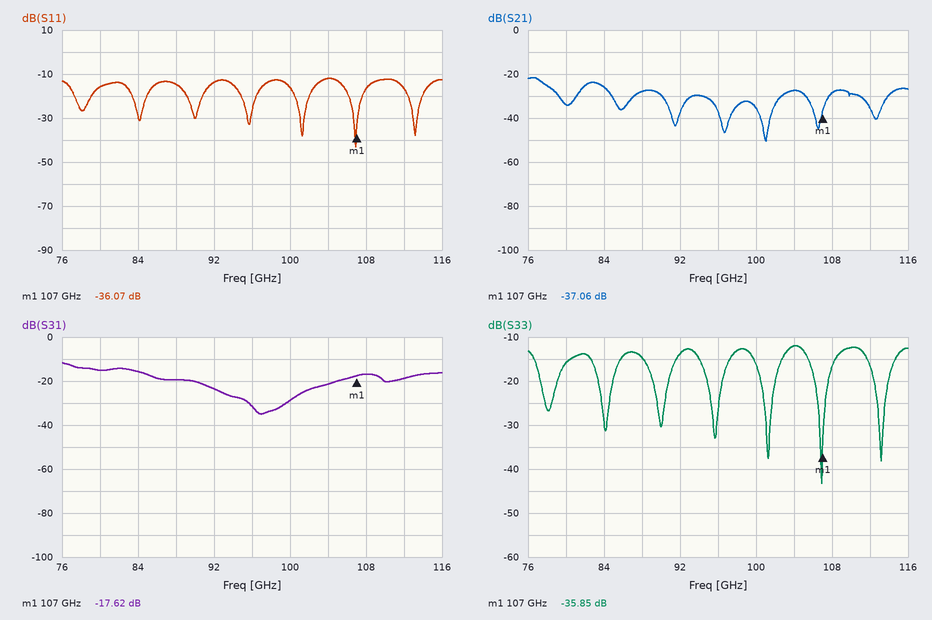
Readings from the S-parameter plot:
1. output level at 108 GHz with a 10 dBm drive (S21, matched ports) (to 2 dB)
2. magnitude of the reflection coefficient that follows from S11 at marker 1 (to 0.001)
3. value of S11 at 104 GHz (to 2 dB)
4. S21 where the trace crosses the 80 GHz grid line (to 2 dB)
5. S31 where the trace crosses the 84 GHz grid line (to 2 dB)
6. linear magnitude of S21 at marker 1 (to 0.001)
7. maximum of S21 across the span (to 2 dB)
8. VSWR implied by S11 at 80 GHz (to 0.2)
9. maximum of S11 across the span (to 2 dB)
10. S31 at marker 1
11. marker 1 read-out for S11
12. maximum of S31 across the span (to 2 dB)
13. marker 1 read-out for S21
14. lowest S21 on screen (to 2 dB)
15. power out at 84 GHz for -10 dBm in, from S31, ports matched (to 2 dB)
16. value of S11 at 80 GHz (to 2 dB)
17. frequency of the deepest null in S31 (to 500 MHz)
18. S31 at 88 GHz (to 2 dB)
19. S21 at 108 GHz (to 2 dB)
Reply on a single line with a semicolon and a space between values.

-18 dBm; 0.016; -12 dB; -34 dB; -16 dB; 0.014; -22 dB; 1.4; -12 dB; -17.62 dB; -36.07 dB; -12 dB; -37.06 dB; -50 dB; -26 dBm; -16 dB; 97.0 GHz; -20 dB; -28 dB
